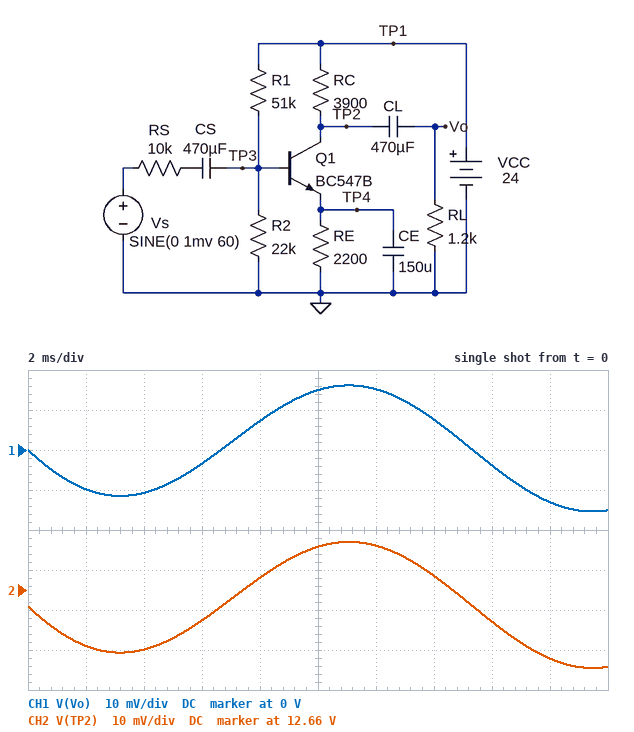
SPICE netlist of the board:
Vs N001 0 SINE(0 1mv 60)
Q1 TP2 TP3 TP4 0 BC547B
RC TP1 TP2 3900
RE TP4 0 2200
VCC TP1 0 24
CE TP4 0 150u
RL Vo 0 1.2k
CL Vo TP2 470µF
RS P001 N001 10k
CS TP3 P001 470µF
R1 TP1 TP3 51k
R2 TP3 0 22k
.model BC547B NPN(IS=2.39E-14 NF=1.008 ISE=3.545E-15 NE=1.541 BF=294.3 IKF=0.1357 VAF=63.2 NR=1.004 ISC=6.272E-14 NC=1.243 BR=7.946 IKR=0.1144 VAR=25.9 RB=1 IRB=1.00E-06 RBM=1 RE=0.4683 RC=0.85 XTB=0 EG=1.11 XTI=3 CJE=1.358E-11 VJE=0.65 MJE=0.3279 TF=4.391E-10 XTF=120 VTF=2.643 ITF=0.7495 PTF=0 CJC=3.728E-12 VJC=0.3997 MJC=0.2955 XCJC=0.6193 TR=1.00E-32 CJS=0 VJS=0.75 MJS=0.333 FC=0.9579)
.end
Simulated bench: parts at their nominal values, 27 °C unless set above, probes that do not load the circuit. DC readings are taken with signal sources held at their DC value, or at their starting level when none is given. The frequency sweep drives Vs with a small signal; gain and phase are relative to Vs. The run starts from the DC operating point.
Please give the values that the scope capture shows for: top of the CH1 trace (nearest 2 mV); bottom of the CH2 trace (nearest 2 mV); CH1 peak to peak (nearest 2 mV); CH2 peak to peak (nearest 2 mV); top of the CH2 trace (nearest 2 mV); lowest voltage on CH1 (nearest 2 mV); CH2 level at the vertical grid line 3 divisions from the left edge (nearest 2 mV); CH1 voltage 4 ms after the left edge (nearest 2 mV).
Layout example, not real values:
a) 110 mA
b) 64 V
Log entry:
a) 16 mV
b) 12.640 V
c) 32 mV
d) 32 mV
e) 12.672 V
f) -16 mV
g) 12.652 V
h) -10 mV
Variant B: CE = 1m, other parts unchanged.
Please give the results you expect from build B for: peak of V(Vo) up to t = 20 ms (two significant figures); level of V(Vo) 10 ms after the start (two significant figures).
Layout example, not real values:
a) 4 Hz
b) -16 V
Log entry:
a) 19 mV
b) 13 mV
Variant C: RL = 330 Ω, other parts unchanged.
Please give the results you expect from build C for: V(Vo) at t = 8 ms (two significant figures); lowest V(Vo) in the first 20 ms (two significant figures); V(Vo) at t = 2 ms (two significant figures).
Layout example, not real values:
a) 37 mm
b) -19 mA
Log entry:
a) 2.5 mV
b) -5.2 mV
c) -3.3 mV
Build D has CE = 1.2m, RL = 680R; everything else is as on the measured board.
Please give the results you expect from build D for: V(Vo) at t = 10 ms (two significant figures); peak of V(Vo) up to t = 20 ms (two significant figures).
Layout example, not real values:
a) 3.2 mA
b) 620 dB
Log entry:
a) 8.0 mV
b) 12 mV
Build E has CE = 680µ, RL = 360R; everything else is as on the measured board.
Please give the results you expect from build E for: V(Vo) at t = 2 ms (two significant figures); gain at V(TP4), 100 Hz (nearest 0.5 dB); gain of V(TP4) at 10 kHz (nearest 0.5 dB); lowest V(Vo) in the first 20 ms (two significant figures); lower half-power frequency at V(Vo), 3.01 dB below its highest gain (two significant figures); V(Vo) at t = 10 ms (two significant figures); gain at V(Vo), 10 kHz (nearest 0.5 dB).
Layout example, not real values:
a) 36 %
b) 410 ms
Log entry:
a) -4.3 mV
b) -26.5 dB
c) -66.5 dB
d) -6.1 mV
e) 7.9 Hz
f) 5.0 mV
g) 16.5 dB
